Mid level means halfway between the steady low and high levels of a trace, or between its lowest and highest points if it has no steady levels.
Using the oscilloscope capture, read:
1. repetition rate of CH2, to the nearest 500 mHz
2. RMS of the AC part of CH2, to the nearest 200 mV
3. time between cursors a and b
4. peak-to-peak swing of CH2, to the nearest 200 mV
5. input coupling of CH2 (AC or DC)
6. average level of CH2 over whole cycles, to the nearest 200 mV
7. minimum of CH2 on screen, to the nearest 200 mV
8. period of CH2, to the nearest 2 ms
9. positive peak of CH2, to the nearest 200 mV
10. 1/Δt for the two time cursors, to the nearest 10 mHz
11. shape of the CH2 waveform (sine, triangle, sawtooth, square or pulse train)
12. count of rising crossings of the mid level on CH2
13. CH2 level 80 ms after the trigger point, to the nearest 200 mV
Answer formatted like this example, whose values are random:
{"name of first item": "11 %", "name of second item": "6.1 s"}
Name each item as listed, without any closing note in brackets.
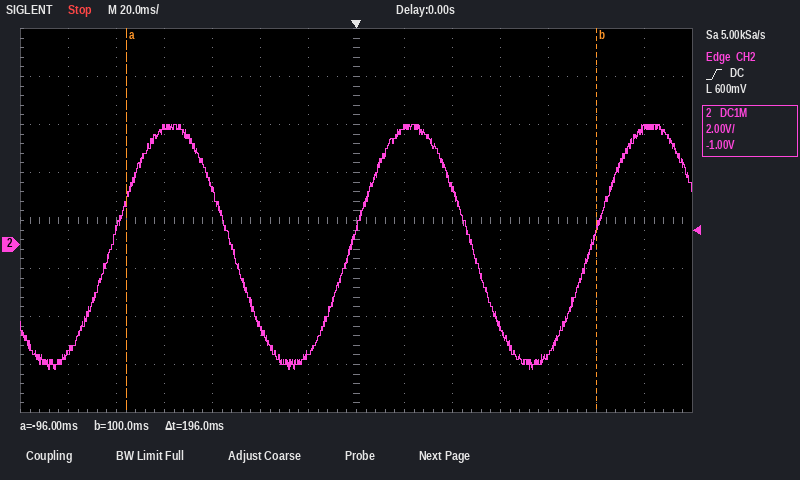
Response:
{"repetition rate of CH2, to the nearest 500 mHz": "10.0 Hz", "RMS of the AC part of CH2, to the nearest 200 mV": "3.6 V", "time between cursors a and b": "196 ms", "peak-to-peak swing of CH2, to the nearest 200 mV": "10.2 V", "input coupling of CH2": "DC", "average level of CH2 over whole cycles, to the nearest 200 mV": "0.0 V", "minimum of CH2 on screen, to the nearest 200 mV": "-5.2 V", "period of CH2, to the nearest 2 ms": "100 ms", "positive peak of CH2, to the nearest 200 mV": "5.0 V", "1/Δt for the two time cursors, to the nearest 10 mHz": "5.10 Hz", "shape of the CH2 waveform": "sine", "count of rising crossings of the mid level on CH2": "3", "CH2 level 80 ms after the trigger point, to the nearest 200 mV": "-4.6 V"}
